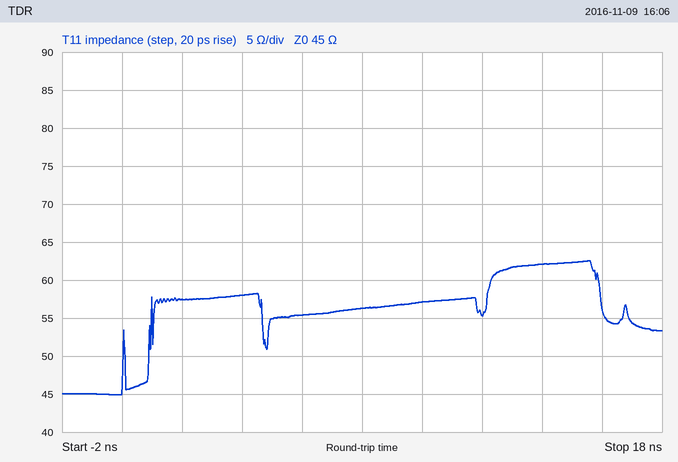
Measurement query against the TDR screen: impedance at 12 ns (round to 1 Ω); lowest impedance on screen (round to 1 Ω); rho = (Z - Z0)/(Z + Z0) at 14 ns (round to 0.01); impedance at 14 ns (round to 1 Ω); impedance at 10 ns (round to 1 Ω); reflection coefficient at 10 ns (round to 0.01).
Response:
55 Ω
45 Ω
+0.16
62 Ω
57 Ω
+0.12
